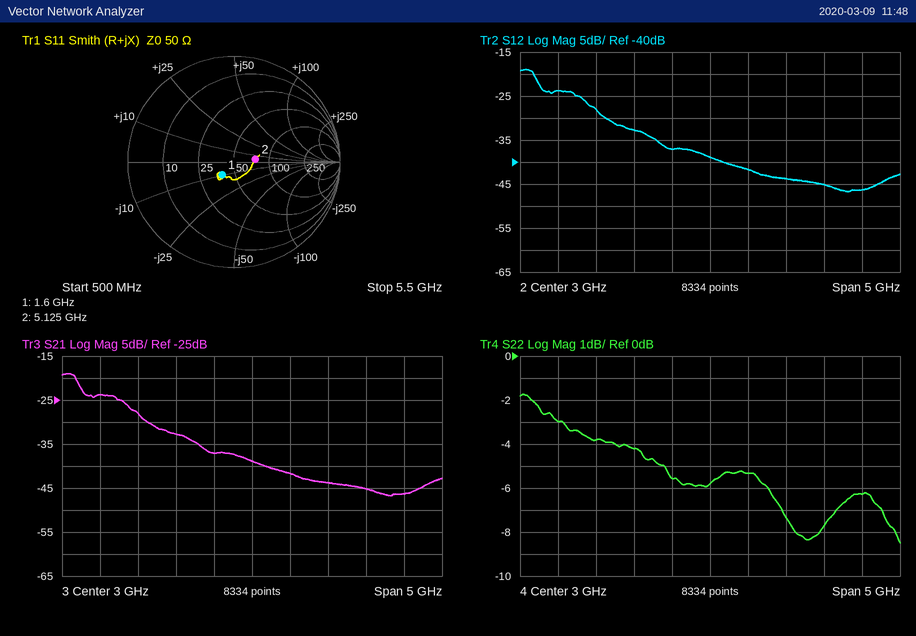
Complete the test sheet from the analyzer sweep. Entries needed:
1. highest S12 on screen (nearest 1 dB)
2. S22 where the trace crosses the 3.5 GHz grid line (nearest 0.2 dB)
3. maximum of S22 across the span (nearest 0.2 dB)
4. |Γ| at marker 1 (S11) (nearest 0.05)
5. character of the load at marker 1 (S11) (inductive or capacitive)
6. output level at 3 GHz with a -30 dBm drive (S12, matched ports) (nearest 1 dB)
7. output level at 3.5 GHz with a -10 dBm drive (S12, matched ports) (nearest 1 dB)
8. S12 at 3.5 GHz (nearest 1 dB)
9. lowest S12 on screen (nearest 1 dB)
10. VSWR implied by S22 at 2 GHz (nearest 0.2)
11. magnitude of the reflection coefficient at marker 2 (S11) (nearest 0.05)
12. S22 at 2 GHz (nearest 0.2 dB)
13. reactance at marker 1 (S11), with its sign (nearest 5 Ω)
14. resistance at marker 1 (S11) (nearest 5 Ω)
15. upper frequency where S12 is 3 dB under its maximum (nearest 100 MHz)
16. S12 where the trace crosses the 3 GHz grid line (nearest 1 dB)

-19 dB
-5.4 dB
-1.8 dB
0.15
capacitive
-69 dBm
-52 dBm
-42 dB
-47 dB
4.2
0.20
-4.2 dB
-10 Ω
40 Ω
700 MHz
-39 dB
